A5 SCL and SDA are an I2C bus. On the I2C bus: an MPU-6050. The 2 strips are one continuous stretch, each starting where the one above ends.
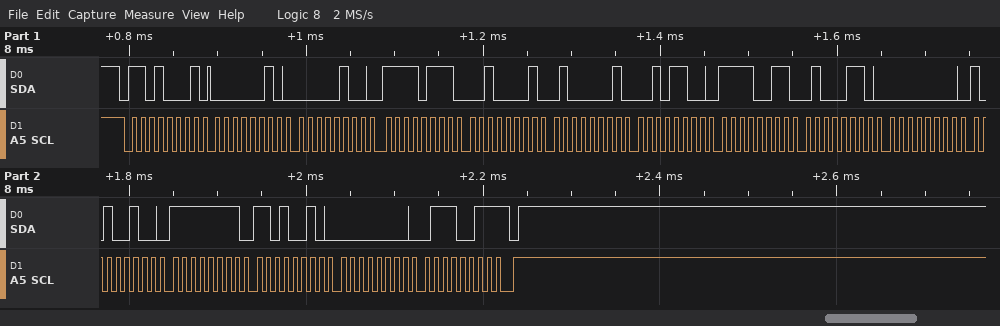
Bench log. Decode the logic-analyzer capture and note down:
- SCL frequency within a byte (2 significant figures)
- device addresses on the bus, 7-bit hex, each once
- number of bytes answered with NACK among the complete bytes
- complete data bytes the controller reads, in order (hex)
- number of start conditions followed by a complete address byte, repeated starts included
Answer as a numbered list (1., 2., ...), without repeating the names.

1. 100 kHz
2. 0x68
3. 1
4. 02 04 F7 21 41 2C F3 46 00 A4 FF D2 00 73
5. 1
